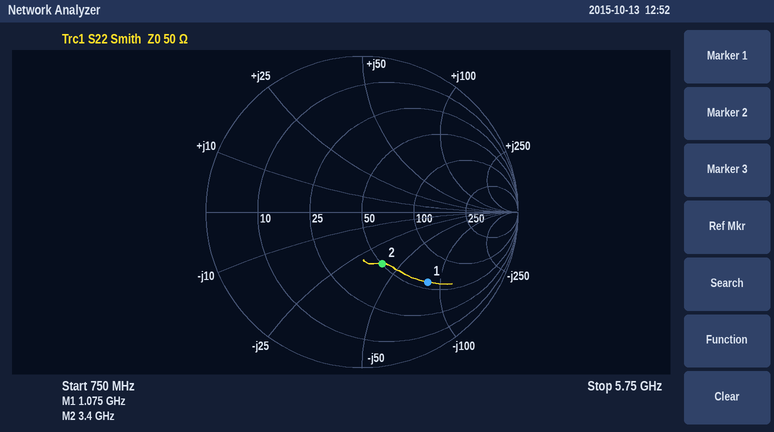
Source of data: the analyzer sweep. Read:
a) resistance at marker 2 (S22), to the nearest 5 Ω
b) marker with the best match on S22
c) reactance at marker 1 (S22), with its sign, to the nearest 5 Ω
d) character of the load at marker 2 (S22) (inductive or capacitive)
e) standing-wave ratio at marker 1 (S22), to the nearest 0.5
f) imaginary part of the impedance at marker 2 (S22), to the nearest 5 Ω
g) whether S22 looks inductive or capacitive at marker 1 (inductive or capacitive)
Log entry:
50 Ω
marker 2
-85 Ω
capacitive
4.0
-40 Ω
capacitive
